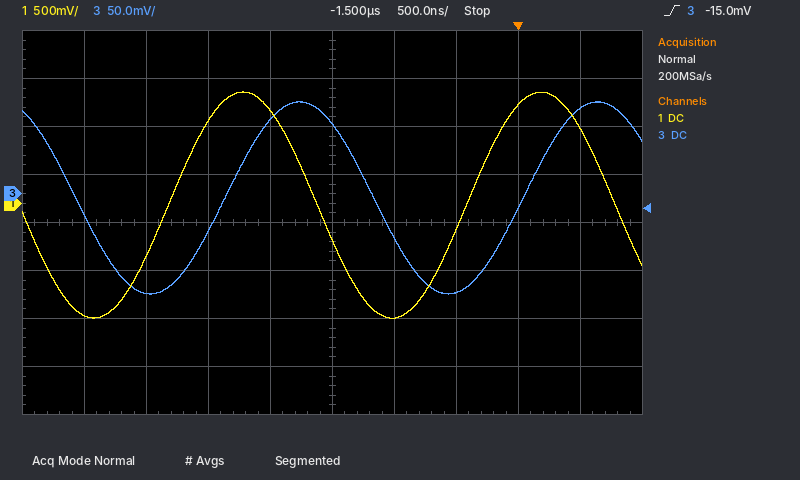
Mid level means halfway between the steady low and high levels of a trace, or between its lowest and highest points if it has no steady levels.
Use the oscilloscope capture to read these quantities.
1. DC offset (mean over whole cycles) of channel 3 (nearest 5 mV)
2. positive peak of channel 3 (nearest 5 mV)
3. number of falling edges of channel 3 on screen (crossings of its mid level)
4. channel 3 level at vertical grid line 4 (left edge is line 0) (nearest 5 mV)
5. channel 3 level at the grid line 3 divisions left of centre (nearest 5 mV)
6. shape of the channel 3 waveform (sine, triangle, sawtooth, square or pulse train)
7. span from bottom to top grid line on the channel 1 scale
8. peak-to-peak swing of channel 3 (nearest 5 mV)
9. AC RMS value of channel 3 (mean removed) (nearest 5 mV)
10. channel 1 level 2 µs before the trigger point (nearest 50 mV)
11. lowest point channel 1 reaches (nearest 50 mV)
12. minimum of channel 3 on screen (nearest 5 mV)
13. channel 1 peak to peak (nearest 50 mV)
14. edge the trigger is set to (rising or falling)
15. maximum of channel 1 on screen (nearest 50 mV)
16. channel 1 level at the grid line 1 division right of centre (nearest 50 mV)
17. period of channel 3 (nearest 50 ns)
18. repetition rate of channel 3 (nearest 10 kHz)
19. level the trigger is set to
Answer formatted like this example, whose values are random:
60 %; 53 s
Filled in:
-5 mV; 95 mV; 2; 75 mV; -105 mV; sine; 4 V; 200 mV; 70 mV; 950 mV; -1.20 V; -105 mV; 2.35 V; rising; 1.15 V; -1.20 V; 2.40 µs; 420 kHz; -15.0 mV
